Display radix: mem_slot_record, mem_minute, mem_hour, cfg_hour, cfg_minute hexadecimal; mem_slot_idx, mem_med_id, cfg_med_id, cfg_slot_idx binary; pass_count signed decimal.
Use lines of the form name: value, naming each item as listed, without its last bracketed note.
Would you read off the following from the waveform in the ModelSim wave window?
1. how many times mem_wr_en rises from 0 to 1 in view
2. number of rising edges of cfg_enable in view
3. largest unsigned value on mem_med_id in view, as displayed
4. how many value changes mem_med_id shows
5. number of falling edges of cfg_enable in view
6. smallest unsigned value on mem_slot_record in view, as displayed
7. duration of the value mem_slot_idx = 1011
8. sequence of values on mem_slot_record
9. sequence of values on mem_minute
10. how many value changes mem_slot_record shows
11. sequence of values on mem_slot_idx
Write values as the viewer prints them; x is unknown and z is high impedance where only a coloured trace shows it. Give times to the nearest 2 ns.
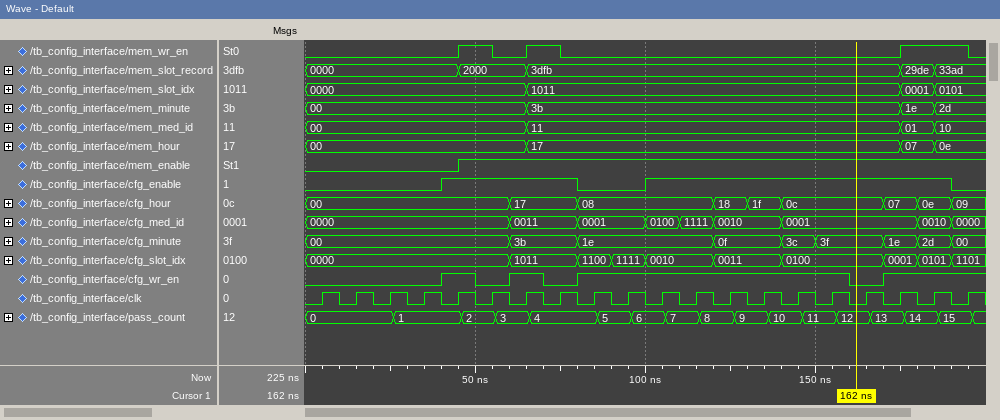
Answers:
how many times mem_wr_en rises from 0 to 1 in view: 3
number of rising edges of cfg_enable in view: 2
largest unsigned value on mem_med_id in view, as displayed: 11
how many value changes mem_med_id shows: 3
number of falling edges of cfg_enable in view: 2
smallest unsigned value on mem_slot_record in view, as displayed: 0000
duration of the value mem_slot_idx = 1011: 110 ns
sequence of values on mem_slot_record: 0000, 2000, 3dfb, 29de, 33ad
sequence of values on mem_minute: 00, 3b, 1e, 2d
how many value changes mem_slot_record shows: 4
sequence of values on mem_slot_idx: 0000, 1011, 0001, 0101
